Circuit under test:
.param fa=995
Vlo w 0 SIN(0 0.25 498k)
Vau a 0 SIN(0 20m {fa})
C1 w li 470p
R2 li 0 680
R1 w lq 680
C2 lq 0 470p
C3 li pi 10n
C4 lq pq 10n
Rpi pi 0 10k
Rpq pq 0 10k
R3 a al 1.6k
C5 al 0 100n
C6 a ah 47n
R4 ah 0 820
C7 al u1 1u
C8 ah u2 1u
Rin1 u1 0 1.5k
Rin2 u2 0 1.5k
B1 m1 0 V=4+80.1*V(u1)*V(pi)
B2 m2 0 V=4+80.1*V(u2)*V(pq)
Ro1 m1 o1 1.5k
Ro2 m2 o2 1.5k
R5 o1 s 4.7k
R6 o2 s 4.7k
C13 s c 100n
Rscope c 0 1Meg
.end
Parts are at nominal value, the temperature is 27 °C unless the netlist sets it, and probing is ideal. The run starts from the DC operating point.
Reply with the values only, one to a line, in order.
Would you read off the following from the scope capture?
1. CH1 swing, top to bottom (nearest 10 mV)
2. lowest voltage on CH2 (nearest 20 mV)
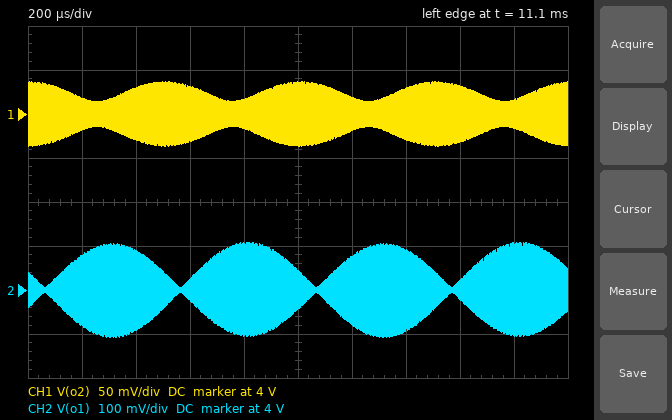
70 mV
3.90 V
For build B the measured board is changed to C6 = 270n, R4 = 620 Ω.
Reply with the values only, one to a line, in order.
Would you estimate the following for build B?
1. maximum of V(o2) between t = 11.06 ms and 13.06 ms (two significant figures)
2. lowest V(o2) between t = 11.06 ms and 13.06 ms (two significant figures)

4.1 V
3.9 V
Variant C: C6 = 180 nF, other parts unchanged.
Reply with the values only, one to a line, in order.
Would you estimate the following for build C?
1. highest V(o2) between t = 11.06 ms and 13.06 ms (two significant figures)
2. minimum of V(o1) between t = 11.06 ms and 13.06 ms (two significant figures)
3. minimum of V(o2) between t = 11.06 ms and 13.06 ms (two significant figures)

4.1 V
3.9 V
3.9 V
